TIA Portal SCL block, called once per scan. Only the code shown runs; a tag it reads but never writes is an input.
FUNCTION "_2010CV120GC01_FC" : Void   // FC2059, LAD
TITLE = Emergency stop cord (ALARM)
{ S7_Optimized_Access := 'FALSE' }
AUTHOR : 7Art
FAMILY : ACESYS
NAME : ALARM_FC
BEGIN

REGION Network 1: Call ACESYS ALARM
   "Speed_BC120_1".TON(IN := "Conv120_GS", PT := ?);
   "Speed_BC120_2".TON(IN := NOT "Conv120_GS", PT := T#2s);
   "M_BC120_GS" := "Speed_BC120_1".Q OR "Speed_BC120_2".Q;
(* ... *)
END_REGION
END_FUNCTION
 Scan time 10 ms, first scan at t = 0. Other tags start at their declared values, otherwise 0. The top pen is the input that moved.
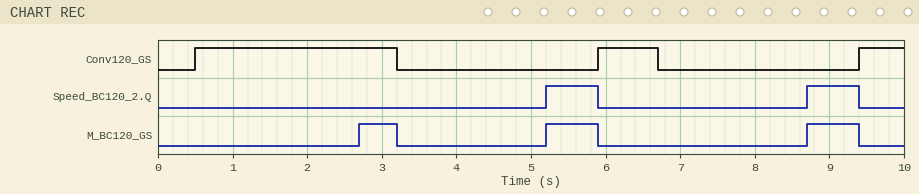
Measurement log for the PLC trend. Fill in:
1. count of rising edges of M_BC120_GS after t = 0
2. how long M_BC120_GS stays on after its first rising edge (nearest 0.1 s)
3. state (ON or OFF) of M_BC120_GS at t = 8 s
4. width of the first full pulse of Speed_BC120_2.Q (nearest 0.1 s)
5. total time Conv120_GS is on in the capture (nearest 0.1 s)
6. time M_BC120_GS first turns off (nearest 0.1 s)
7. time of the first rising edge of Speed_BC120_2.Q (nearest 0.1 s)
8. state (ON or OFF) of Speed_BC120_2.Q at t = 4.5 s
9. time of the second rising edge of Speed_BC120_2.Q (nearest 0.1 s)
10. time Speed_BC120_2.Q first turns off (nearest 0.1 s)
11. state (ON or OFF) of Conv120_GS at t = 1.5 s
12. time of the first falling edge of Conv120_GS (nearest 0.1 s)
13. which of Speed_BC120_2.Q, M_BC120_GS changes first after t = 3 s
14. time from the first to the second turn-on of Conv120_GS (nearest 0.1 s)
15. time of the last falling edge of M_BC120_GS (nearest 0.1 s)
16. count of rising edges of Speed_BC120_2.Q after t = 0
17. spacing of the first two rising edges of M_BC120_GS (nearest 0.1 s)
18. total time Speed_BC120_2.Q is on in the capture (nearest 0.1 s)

3
0.5 s
OFF
0.7 s
4.1 s
3.2 s
5.2 s
OFF
8.7 s
5.9 s
ON
3.2 s
M_BC120_GS
5.4 s
9.4 s
2
2.5 s
1.4 s
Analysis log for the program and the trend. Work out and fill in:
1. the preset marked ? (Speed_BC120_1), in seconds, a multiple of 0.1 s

2.2 s
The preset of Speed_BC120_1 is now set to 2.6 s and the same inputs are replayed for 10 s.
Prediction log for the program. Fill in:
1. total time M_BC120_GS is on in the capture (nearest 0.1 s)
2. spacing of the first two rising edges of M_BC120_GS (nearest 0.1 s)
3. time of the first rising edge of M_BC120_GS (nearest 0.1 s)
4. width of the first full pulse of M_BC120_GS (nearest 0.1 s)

1.5 s
2.1 s
3.1 s
0.1 s
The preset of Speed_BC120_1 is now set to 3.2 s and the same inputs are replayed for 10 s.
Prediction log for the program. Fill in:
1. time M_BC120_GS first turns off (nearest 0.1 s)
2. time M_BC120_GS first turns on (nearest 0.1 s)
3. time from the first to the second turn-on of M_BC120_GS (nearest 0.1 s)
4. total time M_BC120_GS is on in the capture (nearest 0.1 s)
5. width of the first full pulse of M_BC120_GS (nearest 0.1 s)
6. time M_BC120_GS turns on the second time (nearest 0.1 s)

5.9 s
5.2 s
3.5 s
1.4 s
0.7 s
8.7 s
